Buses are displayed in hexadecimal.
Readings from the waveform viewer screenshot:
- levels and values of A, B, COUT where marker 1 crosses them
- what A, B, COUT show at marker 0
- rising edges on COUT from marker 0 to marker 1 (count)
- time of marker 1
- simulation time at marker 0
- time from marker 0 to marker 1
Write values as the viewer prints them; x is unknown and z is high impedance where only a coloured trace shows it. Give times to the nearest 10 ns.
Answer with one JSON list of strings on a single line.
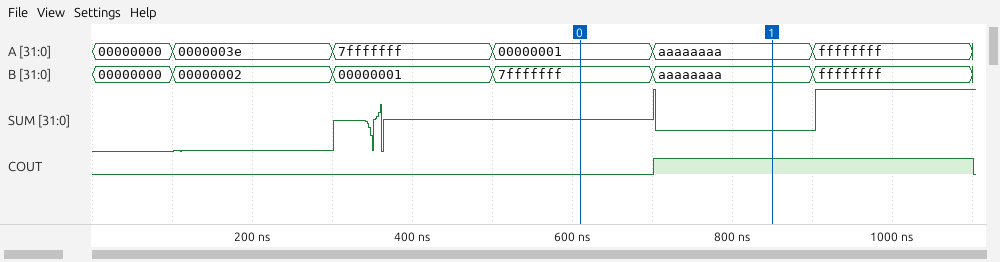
["A=aaaaaaaa, B=aaaaaaaa, COUT=1", "A=00000001, B=7fffffff, COUT=0", "1", "850 ns", "610 ns", "240 ns"]
